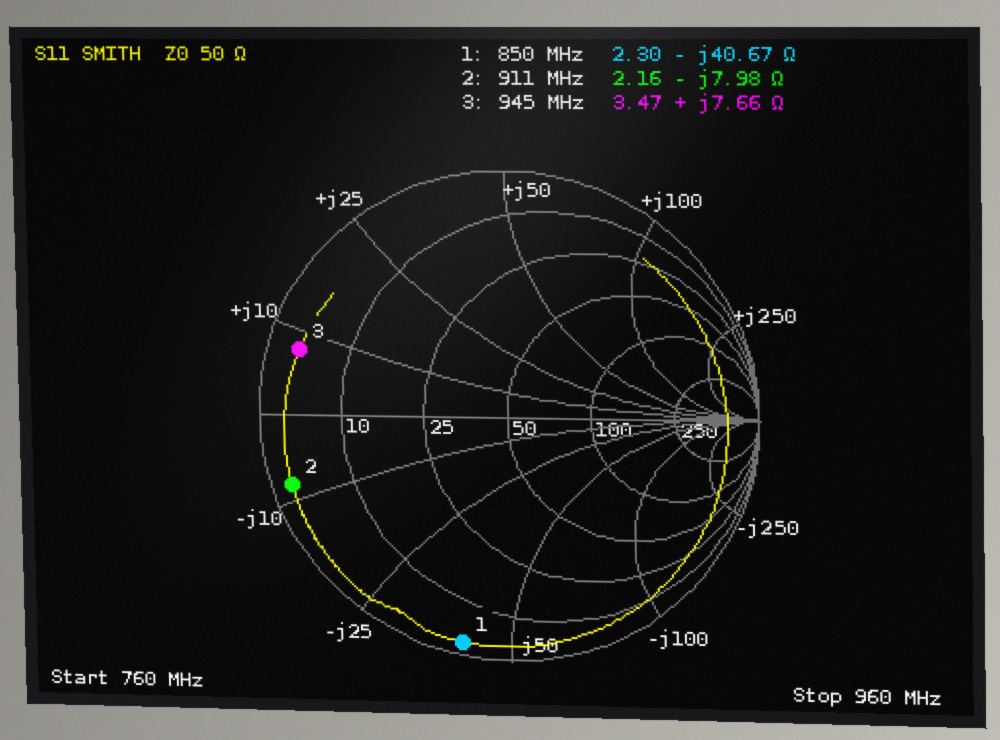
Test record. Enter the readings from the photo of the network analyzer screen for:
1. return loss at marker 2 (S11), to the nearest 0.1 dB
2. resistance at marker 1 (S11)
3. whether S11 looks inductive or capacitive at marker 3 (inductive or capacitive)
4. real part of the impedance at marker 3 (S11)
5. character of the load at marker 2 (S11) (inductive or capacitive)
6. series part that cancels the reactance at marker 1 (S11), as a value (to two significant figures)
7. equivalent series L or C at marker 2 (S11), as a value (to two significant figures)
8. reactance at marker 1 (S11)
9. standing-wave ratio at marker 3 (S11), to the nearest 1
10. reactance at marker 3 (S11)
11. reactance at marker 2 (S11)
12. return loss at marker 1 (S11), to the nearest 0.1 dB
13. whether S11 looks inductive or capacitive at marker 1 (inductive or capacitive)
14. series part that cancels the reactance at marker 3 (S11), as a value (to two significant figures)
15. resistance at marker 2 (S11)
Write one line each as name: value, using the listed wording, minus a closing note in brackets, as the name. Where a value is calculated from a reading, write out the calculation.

return loss at marker 2 (S11), to the nearest 0.1 dB: 0.7 dB
resistance at marker 1: 2.30 Ω
whether S11 looks inductive or capacitive at marker 3: inductive
real part of the impedance at marker 3: 3.47 Ω
character of the load at marker 2 (S11): capacitive
series part that cancels the reactance at marker 1 (S11), as a value: L = 40.67 Ω/(2π × 850 MHz) ≈ 7.6 nH
equivalent series L or C at marker 2 (S11), as a value: C = 1/(2π × 911 MHz × 7.98 Ω) ≈ 22 pF
reactance at marker 1: -40.67 Ω
standing-wave ratio at marker 3 (S11), to the nearest 1: 15
reactance at marker 3: +7.66 Ω
reactance at marker 2: -7.98 Ω
return loss at marker 1 (S11), to the nearest 0.1 dB: 0.5 dB
whether S11 looks inductive or capacitive at marker 1: capacitive
series part that cancels the reactance at marker 3 (S11), as a value: C = 1/(2π × 945 MHz × 7.66 Ω) ≈ 22 pF
resistance at marker 2: 2.16 Ω
